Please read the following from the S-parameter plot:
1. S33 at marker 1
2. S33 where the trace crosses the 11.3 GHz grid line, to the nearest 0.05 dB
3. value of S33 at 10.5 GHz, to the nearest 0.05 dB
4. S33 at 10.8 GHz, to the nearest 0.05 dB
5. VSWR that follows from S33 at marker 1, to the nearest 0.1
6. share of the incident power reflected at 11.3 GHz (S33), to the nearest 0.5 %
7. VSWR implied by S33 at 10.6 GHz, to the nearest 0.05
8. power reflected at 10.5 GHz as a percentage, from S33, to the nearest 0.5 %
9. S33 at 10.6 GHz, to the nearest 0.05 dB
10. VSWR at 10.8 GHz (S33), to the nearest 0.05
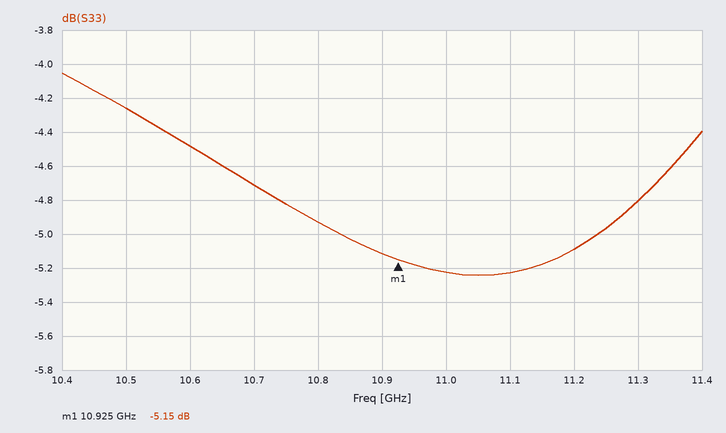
-5.15 dB
-4.80 dB
-4.25 dB
-4.95 dB
3.5
33.0 %
3.95
37.5 %
-4.50 dB
3.60
